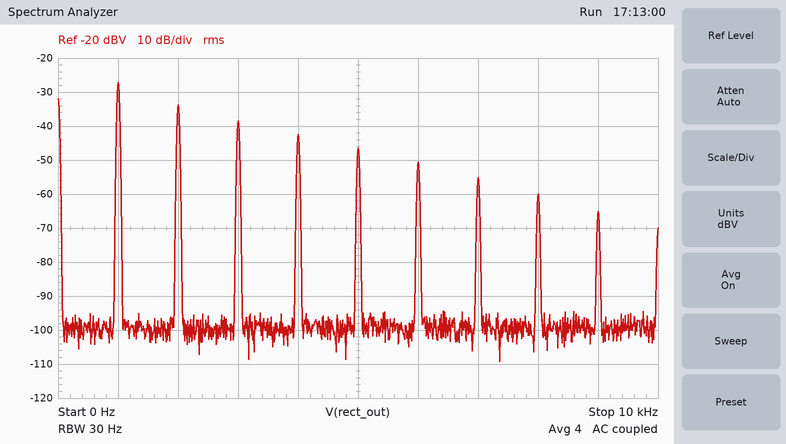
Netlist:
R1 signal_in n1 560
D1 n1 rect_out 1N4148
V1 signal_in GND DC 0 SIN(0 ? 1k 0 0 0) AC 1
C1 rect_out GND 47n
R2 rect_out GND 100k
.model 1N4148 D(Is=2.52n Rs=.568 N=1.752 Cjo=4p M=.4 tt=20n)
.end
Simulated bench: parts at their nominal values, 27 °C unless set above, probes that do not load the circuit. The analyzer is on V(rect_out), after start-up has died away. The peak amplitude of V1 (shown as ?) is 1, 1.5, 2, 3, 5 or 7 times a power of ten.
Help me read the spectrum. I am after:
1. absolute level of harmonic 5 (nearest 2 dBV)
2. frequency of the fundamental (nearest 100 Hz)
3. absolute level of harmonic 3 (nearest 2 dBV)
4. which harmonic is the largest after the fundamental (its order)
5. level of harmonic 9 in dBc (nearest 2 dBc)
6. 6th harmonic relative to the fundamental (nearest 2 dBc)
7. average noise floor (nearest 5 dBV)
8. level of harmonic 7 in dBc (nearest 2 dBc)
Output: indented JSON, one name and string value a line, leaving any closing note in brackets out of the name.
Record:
{
  "absolute level of harmonic 5": "-46 dBV",
  "frequency of the fundamental": "1.0 kHz",
  "absolute level of harmonic 3": "-38 dBV",
  "which harmonic is the largest after the fundamental": "2",
  "level of harmonic 9 in dBc": "-38 dBc",
  "6th harmonic relative to the fundamental": "-24 dBc",
  "average noise floor": "-100 dBV",
  "level of harmonic 7 in dBc": "-28 dBc"
}
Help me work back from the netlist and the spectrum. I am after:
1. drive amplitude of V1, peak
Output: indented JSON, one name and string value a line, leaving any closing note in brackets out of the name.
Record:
{
  "drive amplitude of V1, peak": "1.5 V"
}
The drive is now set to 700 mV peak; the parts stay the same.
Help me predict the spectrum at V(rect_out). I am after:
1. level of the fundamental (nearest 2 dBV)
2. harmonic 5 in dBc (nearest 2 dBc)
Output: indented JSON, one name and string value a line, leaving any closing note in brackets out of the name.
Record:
{
  "level of the fundamental": "-38 dBV",
  "harmonic 5 in dBc": "-22 dBc"
}
